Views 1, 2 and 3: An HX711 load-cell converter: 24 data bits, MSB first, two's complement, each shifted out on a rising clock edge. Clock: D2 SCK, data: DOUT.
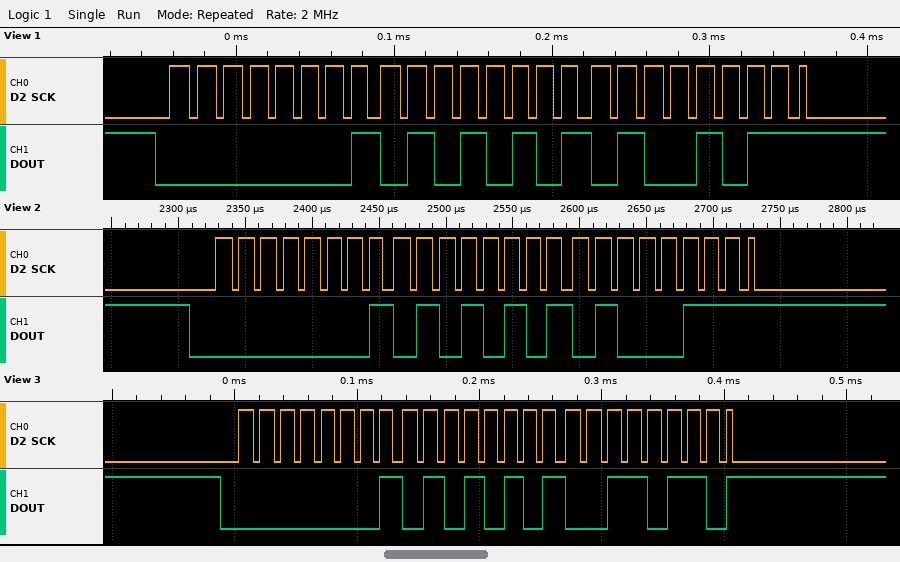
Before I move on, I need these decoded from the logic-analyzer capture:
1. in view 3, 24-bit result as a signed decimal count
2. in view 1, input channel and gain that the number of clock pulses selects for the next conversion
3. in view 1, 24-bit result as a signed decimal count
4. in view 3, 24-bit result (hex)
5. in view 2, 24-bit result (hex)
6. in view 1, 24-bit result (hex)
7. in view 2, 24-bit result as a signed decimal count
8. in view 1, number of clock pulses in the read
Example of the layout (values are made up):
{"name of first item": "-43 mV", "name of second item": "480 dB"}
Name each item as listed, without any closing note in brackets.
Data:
{"in view 3, 24-bit result as a signed decimal count": "87350", "in view 1, input channel and gain that the number of clock pulses selects for the next conversion": "channel A, gain 128", "in view 1, 24-bit result as a signed decimal count": "87371", "in view 3, 24-bit result": "0x015536", "in view 2, 24-bit result": "0x015547", "in view 1, 24-bit result": "0x01554B", "in view 2, 24-bit result as a signed decimal count": "87367", "in view 1, number of clock pulses in the read": "25"}
